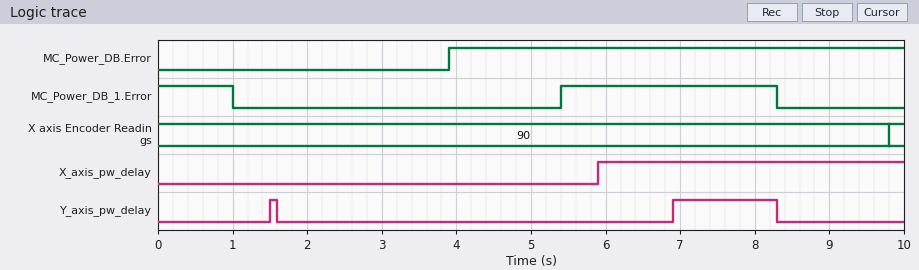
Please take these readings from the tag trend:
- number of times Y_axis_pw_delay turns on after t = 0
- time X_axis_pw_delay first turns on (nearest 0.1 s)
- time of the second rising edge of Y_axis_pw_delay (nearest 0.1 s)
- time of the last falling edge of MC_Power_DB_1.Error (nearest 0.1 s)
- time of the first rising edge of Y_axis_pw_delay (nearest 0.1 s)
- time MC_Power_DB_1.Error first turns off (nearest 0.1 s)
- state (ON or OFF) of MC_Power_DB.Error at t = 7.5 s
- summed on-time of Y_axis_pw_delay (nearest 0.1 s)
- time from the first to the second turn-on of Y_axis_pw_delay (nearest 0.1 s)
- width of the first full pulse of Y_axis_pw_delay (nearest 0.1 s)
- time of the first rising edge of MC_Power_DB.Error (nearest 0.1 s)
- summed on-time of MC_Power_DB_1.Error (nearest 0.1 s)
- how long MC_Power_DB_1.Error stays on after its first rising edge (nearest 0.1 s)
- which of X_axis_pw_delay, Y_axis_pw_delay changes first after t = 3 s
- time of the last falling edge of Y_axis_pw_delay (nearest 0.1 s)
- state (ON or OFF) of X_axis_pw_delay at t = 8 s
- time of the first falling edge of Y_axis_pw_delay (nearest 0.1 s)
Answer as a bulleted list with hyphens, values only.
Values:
- 2
- 5.9 s
- 6.9 s
- 8.3 s
- 1.5 s
- 1.0 s
- ON
- 1.5 s
- 5.4 s
- 0.1 s
- 3.9 s
- 3.9 s
- 2.9 s
- X_axis_pw_delay
- 8.3 s
- ON
- 1.6 s
